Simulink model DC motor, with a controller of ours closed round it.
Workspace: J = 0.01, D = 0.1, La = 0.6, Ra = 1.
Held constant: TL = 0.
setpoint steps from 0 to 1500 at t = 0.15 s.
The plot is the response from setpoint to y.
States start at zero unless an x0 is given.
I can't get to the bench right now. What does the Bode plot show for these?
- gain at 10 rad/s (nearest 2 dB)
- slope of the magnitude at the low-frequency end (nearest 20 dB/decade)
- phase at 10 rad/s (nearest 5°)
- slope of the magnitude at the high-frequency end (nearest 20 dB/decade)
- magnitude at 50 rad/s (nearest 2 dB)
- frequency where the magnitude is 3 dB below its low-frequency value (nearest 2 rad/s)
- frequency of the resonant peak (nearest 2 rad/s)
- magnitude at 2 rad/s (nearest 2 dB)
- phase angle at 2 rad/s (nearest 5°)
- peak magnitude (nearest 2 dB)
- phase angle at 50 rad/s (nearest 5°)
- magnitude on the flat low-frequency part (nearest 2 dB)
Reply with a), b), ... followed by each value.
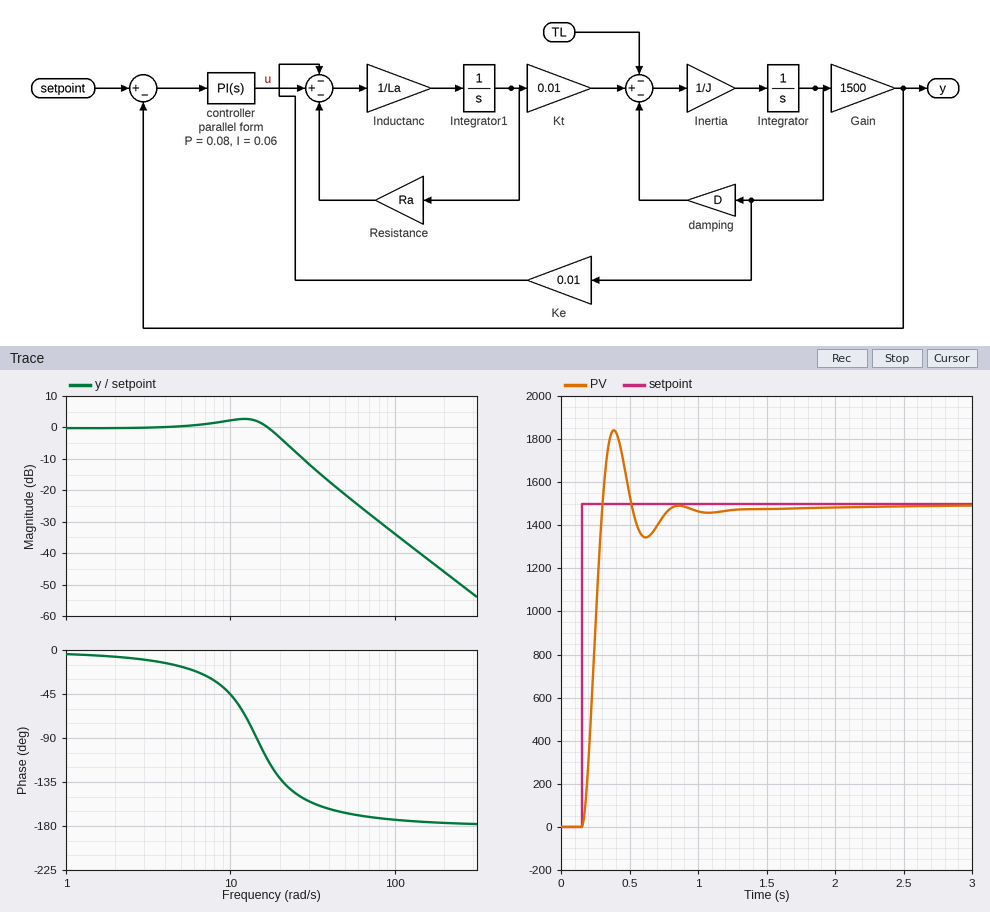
a) 2 dB
b) 0 dB/decade
c) -45°
d) -40 dB/decade
e) -22 dB
f) 20 rad/s
g) 12 rad/s
h) 0 dB
i) -5°
j) 2 dB
k) -165°
l) 0 dB
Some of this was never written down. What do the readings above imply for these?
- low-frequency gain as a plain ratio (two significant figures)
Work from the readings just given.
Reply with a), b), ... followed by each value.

a) 1.0
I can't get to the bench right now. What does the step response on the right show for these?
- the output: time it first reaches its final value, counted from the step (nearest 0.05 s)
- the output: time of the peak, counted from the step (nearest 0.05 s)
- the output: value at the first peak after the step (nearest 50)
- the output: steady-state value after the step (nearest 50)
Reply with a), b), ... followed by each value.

a) 0.15 s
b) 0.25 s
c) 1850
d) 1500
